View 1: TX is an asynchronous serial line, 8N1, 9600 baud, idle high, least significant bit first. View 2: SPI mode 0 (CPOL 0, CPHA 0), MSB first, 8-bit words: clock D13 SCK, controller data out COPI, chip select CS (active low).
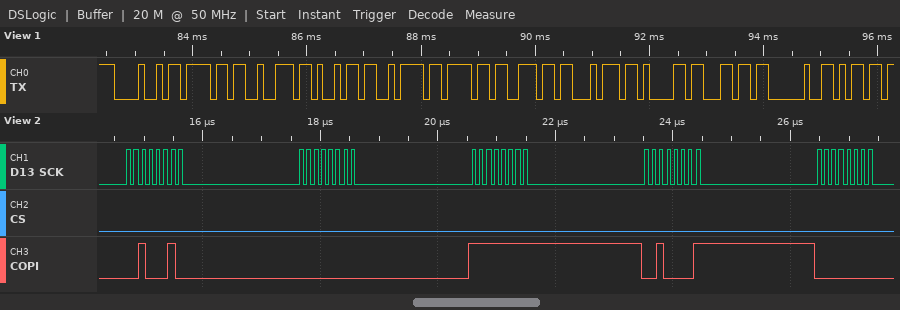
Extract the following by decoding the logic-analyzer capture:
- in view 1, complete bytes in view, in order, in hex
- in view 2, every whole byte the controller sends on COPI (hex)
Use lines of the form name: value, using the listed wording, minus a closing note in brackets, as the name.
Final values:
in view 1, complete bytes in view, in order, in hex: 48 6F 72 69 7A 6F 6E 74 61 6C 20 6D
in view 2, every whole byte the controller sends on COPI: 22 00 FF 21 00
